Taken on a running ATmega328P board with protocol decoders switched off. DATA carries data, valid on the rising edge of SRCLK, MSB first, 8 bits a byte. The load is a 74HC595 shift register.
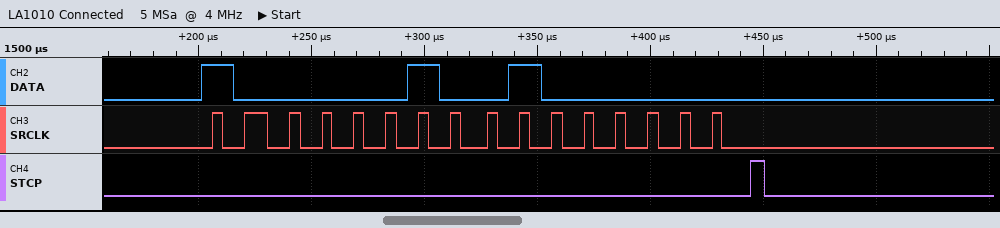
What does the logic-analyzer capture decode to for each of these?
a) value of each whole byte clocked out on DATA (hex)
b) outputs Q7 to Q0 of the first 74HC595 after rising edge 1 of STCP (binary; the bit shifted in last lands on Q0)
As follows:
82 40
01000000
